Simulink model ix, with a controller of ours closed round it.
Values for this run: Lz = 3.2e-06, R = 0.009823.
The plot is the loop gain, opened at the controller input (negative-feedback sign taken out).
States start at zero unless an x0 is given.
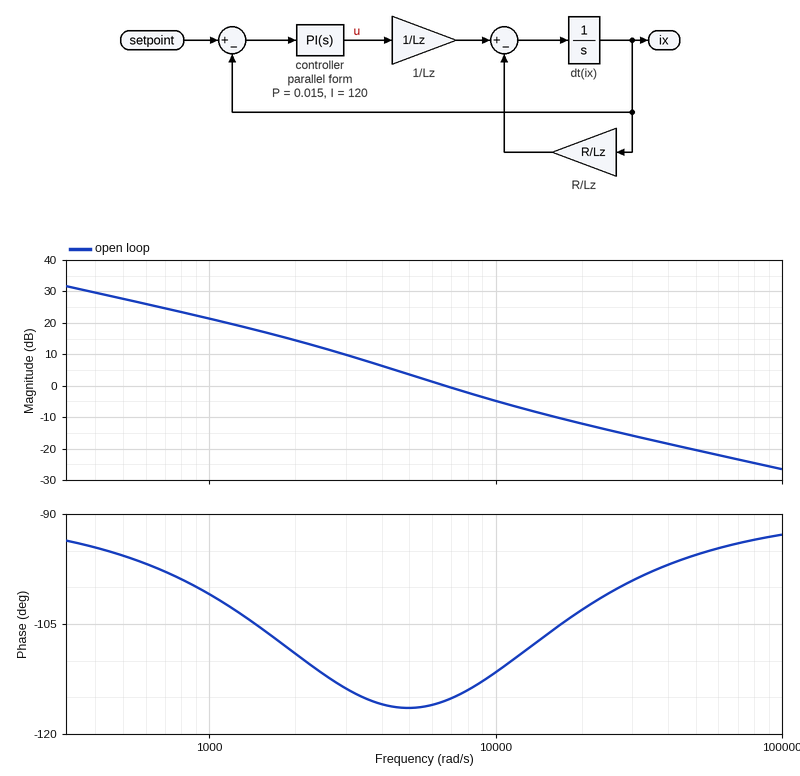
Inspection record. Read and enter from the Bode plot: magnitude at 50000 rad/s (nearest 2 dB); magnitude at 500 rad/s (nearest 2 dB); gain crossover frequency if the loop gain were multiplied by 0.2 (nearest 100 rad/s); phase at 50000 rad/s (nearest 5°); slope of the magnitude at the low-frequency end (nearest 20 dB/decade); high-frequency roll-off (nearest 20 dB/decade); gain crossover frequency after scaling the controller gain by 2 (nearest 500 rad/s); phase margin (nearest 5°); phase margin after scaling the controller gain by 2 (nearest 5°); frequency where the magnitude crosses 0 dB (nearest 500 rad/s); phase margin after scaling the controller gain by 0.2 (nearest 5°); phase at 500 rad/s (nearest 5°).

-20 dB
28 dB
2100 rad/s
-95°
-20 dB/decade
-20 dB/decade
11000 rad/s
65°
70°
6500 rad/s
70°
-95°
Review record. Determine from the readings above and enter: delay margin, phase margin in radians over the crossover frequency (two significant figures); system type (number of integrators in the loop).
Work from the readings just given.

0.00017 s
1
